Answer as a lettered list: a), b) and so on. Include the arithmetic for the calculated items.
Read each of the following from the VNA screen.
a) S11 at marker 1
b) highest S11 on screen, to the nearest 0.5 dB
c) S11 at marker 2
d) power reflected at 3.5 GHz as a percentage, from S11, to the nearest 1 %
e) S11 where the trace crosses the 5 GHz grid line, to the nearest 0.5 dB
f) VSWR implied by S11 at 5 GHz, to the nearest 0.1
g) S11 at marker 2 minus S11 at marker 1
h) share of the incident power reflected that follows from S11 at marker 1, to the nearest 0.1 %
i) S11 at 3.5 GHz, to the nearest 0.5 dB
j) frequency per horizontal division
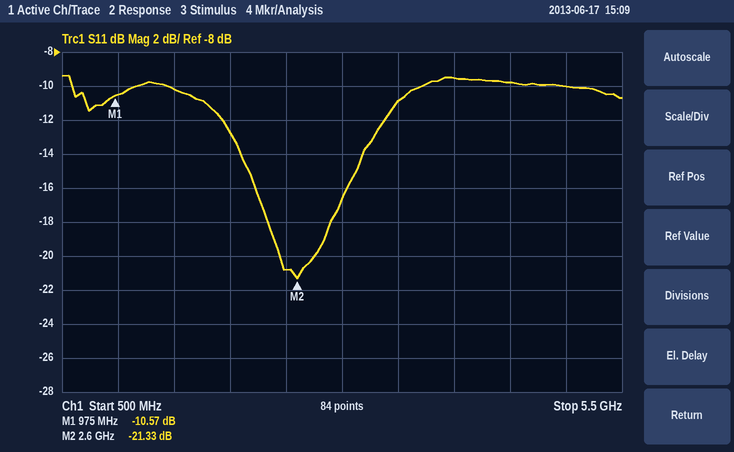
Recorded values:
a) -10.57 dB
b) -9.5 dB
c) -21.33 dB
d) 10^(-11/10) ≈ 8 %
e) -10.0 dB
f) |Γ| = 10^(-10/20) = 0.3162; VSWR = (1 + 0.3162)/(1 − 0.3162) ≈ 1.9
g) -21.33 − (-10.57) = -10.76 dB
h) 10^(-10.57/10) ≈ 8.8 %
i) -11.0 dB
j) 500 MHz
